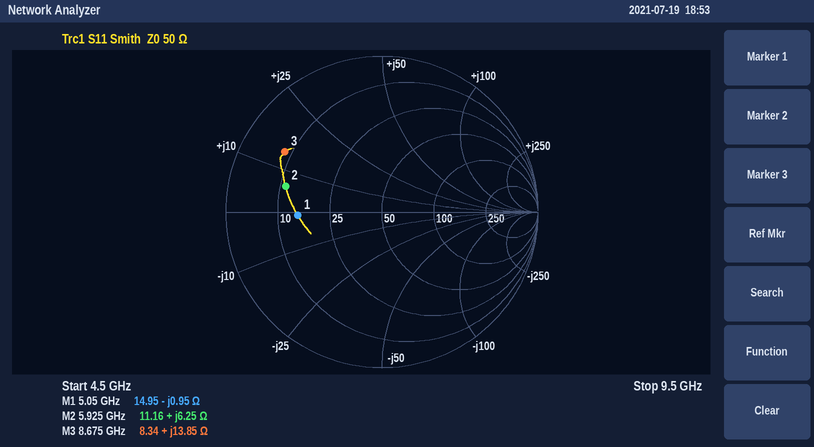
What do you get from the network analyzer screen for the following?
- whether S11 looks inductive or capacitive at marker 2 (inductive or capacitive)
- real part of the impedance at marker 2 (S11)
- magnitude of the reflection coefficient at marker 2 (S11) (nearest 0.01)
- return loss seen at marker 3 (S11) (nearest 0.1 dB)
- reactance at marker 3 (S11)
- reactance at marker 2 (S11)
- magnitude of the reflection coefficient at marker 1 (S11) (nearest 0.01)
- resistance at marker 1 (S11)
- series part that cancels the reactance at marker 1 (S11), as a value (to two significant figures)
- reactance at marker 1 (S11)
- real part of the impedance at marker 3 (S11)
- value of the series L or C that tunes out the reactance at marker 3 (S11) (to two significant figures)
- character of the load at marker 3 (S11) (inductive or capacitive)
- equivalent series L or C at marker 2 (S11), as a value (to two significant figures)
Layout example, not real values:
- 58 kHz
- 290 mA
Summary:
- inductive
- 11.16 Ω
- 0.64
- 2.7 dB
- +13.85 Ω
- +6.25 Ω
- 0.54
- 14.95 Ω
- 30 pH
- -0.95 Ω
- 8.34 Ω
- 1.3 pF
- inductive
- 170 pH
